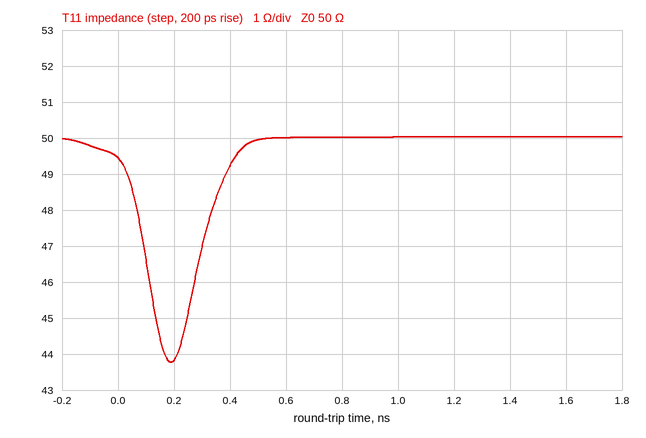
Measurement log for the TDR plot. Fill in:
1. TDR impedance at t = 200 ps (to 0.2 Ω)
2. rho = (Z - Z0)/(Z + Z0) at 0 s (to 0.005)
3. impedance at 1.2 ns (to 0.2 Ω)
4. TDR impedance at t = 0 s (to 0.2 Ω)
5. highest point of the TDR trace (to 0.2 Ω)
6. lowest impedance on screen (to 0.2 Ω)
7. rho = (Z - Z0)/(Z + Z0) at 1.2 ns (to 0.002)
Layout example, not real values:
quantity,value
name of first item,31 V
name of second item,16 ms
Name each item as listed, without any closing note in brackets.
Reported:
quantity,value
TDR impedance at t = 200 ps,43.8 Ω
rho = (Z - Z0)/(Z + Z0) at 0 s,-0.005
impedance at 1.2 ns,50.0 Ω
TDR impedance at t = 0 s,49.4 Ω
highest point of the TDR trace,50.0 Ω
lowest impedance on screen,43.8 Ω
rho = (Z - Z0)/(Z + Z0) at 1.2 ns,0.000
